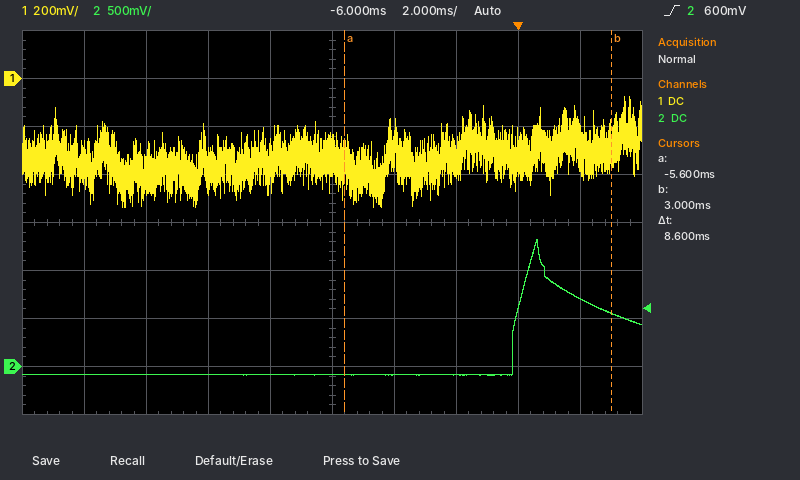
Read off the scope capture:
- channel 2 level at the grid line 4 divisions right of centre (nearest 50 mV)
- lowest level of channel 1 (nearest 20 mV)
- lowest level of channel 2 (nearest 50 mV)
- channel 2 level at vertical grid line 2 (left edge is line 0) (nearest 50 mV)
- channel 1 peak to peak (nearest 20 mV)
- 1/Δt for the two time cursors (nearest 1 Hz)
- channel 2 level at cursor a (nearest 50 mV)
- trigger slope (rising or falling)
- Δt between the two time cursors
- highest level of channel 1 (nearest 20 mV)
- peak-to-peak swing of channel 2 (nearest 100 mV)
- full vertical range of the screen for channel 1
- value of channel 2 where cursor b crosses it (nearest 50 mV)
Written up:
700 mV
-540 mV
-100 mV
-100 mV
460 mV
116 Hz
-100 mV
rising
8.6 ms
-80 mV
1.40 V
1.6 V
550 mV
